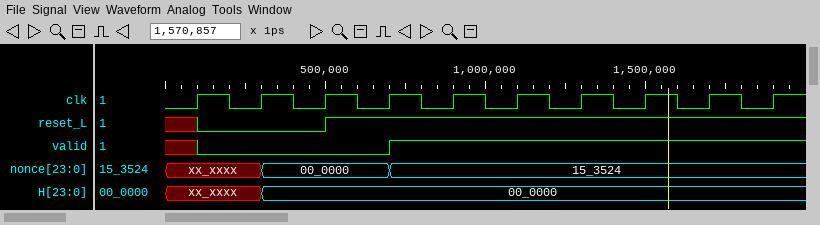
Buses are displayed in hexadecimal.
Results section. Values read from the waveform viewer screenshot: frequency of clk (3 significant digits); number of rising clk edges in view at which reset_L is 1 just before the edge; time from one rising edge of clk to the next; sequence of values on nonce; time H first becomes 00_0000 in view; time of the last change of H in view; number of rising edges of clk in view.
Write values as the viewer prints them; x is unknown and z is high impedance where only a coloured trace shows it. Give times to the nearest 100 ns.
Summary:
5.00 MHz
7
200 ns
xx_xxxx, 00_0000, 15_3524
300 ns
300 ns
10
